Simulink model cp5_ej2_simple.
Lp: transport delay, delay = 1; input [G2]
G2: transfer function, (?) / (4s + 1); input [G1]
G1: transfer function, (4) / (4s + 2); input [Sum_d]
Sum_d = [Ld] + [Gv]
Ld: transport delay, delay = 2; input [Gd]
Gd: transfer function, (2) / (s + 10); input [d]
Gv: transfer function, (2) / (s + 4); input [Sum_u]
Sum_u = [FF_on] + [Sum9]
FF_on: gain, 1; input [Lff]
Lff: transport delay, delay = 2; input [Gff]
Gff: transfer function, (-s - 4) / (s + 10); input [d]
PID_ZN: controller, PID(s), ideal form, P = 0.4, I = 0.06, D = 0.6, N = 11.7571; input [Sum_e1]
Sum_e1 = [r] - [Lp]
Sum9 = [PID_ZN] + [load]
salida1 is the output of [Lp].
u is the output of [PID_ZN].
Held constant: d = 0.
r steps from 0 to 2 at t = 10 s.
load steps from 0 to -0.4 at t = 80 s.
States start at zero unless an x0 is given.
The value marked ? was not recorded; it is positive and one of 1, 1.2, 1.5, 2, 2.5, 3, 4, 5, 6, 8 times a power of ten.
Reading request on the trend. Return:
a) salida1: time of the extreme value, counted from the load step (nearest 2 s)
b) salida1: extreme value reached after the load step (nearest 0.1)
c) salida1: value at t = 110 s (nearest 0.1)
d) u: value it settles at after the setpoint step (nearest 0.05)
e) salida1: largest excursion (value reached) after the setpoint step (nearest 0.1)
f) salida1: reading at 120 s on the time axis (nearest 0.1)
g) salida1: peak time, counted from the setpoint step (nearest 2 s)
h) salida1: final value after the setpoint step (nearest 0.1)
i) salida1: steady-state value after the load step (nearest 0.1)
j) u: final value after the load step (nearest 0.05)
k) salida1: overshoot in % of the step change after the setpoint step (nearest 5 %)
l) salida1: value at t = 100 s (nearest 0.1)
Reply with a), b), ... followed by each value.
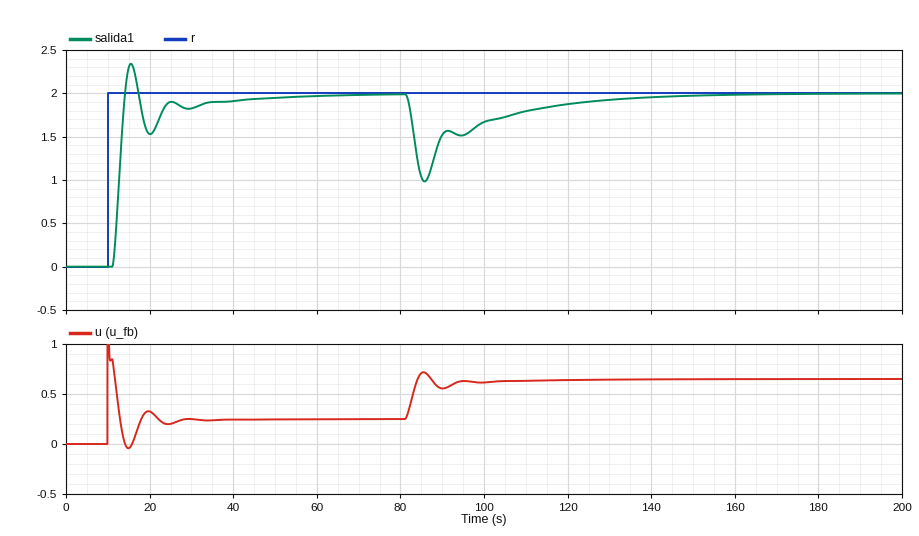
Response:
a) 6 s
b) 1.0
c) 1.8
d) 0.25
e) 2.3
f) 1.9
g) 6 s
h) 2.0
i) 2.0
j) 0.65
k) 15 %
l) 1.7
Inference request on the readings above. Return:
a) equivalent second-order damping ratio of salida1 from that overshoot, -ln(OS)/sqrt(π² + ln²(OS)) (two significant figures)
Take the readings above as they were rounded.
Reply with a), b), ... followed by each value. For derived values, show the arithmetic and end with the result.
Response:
a) ln(0.15) = -1.897; 1.897 / sqrt(9.870 + 3.599) = 0.52
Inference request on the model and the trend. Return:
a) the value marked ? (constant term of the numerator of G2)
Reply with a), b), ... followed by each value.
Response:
a) 8
